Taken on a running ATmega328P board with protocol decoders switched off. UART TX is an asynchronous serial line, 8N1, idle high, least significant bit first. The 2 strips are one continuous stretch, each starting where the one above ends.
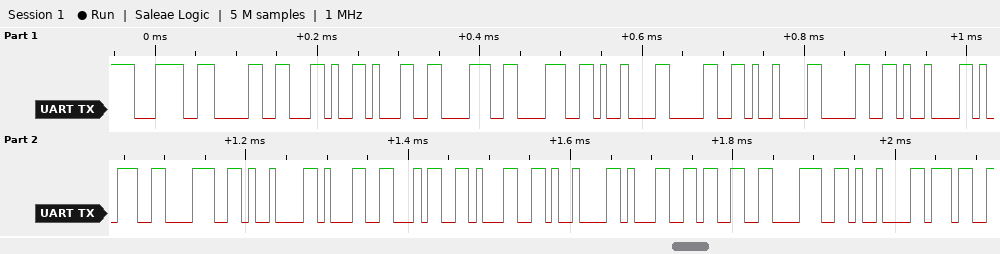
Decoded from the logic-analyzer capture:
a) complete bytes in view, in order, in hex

3C 30 2C 31 38 38 09 30 09 30 09 39 38 09 31 34 31 09 31 33 38 09 37
